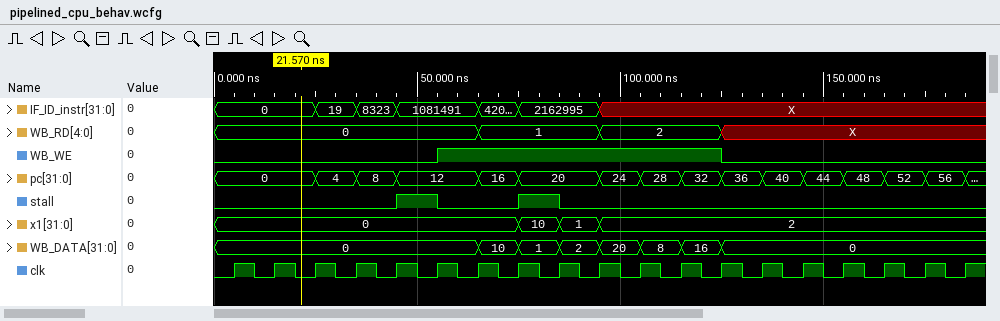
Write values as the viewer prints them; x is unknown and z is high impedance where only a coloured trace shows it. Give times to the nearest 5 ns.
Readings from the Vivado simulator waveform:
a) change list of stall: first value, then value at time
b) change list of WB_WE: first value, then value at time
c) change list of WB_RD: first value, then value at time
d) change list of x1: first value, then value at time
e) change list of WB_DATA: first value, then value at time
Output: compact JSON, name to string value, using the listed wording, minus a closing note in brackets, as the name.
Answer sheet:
{"change list of stall: first value, then value at time": "0, 1 at 45 ns, 0 at 55 ns, 1 at 75 ns, 0 at 85 ns", "change list of WB_WE: first value, then value at time": "0, 1 at 55 ns, 0 at 125 ns", "change list of WB_RD: first value, then value at time": "0, 1 at 65 ns, 2 at 95 ns, X at 125 ns", "change list of x1: first value, then value at time": "0, 10 at 75 ns, 1 at 85 ns, 2 at 95 ns", "change list of WB_DATA: first value, then value at time": "0, 10 at 65 ns, 1 at 75 ns, 2 at 85 ns, 20 at 95 ns, 8 at 105 ns, 16 at 115 ns, 0 at 125 ns"}
